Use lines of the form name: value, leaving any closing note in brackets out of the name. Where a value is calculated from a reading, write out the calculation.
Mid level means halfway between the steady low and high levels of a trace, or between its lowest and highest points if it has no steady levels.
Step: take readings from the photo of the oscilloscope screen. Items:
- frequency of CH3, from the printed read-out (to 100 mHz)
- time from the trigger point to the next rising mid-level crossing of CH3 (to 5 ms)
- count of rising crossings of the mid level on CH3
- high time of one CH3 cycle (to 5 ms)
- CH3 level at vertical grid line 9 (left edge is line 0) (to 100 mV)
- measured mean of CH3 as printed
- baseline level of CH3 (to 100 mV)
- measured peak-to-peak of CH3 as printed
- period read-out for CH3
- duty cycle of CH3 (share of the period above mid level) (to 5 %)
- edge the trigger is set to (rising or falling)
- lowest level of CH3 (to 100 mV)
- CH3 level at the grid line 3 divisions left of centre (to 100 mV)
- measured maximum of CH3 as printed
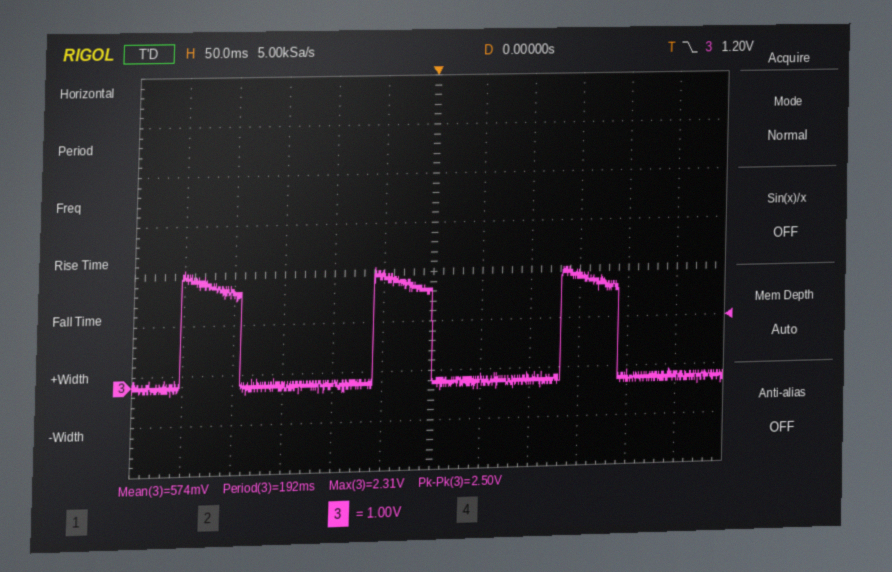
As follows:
frequency of CH3, from the printed read-out: 1 / 192 ms ≈ 5.2 Hz
time from the trigger point to the next rising mid-level crossing of CH3: 130 ms
count of rising crossings of the mid level on CH3: 3
high time of one CH3 cycle: 60 ms
CH3 level at vertical grid line 9 (left edge is line 0): 2.1 V
measured mean of CH3 as printed: 574 mV
baseline level of CH3: 0.0 V
measured peak-to-peak of CH3 as printed: 2.50 V
period read-out for CH3: 192 ms
duty cycle of CH3 (share of the period above mid level): 30 %
edge the trigger is set to: falling
lowest level of CH3: -200 mV
CH3 level at the grid line 3 divisions left of centre: 0.0 V
measured maximum of CH3 as printed: 2.31 V
